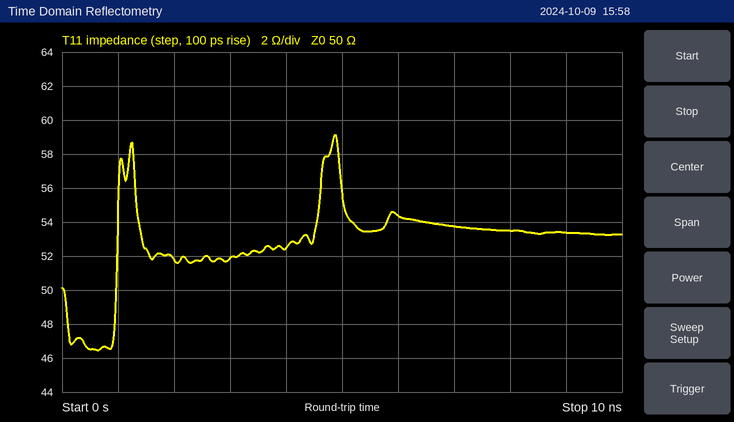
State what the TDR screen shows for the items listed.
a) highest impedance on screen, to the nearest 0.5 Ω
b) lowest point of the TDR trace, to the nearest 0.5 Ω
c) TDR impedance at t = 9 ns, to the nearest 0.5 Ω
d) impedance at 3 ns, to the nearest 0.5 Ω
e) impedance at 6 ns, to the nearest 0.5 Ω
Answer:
59.0 Ω
46.5 Ω
53.5 Ω
52.0 Ω
54.5 Ω
